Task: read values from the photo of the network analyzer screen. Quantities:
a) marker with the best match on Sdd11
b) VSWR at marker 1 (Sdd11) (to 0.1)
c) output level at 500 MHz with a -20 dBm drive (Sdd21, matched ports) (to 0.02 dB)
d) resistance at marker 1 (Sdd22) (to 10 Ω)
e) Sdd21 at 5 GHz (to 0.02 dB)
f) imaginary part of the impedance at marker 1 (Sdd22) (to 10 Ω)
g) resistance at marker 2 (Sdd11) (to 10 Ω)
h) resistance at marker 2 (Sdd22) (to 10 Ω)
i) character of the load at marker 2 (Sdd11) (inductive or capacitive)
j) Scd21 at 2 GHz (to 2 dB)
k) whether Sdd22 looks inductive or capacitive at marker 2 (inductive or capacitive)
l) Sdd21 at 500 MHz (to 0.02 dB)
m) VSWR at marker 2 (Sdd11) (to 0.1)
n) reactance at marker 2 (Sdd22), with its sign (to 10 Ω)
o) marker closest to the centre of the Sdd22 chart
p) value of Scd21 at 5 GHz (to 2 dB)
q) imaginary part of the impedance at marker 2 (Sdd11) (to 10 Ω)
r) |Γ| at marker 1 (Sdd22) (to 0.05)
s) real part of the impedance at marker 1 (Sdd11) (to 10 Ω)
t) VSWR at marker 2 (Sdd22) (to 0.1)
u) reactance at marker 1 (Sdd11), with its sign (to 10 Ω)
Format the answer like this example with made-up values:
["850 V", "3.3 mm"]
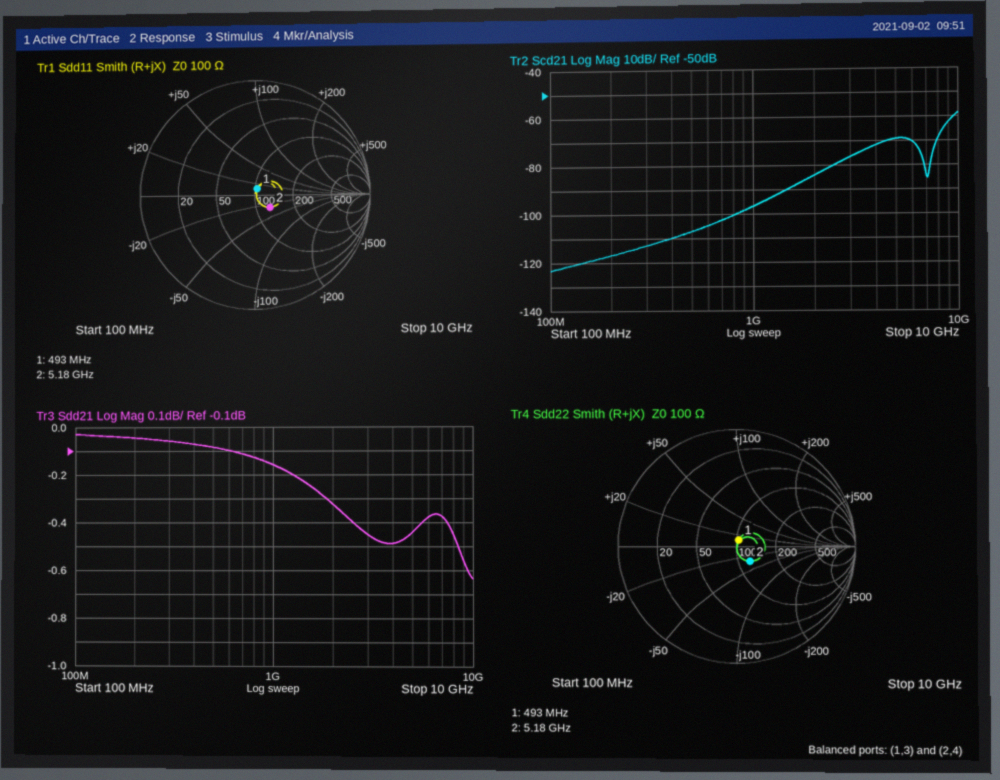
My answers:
["marker 1", "1.1", "-20.08 dBm", "100 Ω", "-0.44 dB", "+10 Ω", "130 Ω", "120 Ω", "capacitive", "-84 dB", "capacitive", "-0.08 dB", "1.4", "-30 Ω", "marker 1", "-70 dB", "-30 Ω", "0.05", "100 Ω", "1.4", "+10 Ω"]
